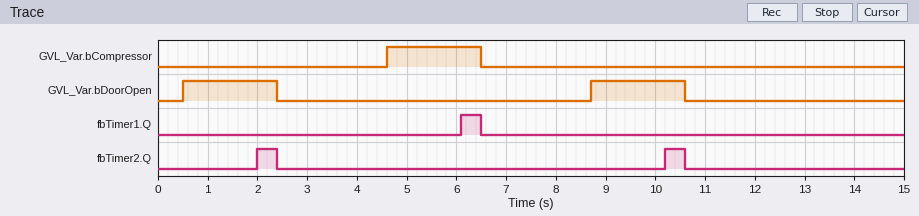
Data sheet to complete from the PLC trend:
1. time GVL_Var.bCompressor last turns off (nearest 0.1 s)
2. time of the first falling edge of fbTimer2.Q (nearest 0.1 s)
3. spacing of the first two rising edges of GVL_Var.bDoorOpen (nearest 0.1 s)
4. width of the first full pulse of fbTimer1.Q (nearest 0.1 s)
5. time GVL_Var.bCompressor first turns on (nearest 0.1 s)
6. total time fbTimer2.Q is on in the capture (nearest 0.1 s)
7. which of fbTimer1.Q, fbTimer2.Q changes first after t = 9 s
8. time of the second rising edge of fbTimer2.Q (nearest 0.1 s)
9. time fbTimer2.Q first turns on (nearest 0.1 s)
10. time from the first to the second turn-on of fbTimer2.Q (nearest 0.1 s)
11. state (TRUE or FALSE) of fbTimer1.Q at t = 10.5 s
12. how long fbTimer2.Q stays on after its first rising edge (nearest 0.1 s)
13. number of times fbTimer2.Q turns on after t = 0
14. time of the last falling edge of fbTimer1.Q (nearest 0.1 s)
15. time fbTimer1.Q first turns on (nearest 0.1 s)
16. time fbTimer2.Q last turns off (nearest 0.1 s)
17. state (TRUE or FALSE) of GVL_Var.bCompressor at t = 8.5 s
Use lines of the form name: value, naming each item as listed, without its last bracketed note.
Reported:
time GVL_Var.bCompressor last turns off: 6.5 s
time of the first falling edge of fbTimer2.Q: 2.4 s
spacing of the first two rising edges of GVL_Var.bDoorOpen: 8.2 s
width of the first full pulse of fbTimer1.Q: 0.4 s
time GVL_Var.bCompressor first turns on: 4.6 s
total time fbTimer2.Q is on in the capture: 0.8 s
which of fbTimer1.Q, fbTimer2.Q changes first after t = 9 s: fbTimer2.Q
time of the second rising edge of fbTimer2.Q: 10.2 s
time fbTimer2.Q first turns on: 2.0 s
time from the first to the second turn-on of fbTimer2.Q: 8.2 s
state (TRUE or FALSE) of fbTimer1.Q at t = 10.5 s: FALSE
how long fbTimer2.Q stays on after its first rising edge: 0.4 s
number of times fbTimer2.Q turns on after t = 0: 2
time of the last falling edge of fbTimer1.Q: 6.5 s
time fbTimer1.Q first turns on: 6.1 s
time fbTimer2.Q last turns off: 10.6 s
state (TRUE or FALSE) of GVL_Var.bCompressor at t = 8.5 s: FALSE
